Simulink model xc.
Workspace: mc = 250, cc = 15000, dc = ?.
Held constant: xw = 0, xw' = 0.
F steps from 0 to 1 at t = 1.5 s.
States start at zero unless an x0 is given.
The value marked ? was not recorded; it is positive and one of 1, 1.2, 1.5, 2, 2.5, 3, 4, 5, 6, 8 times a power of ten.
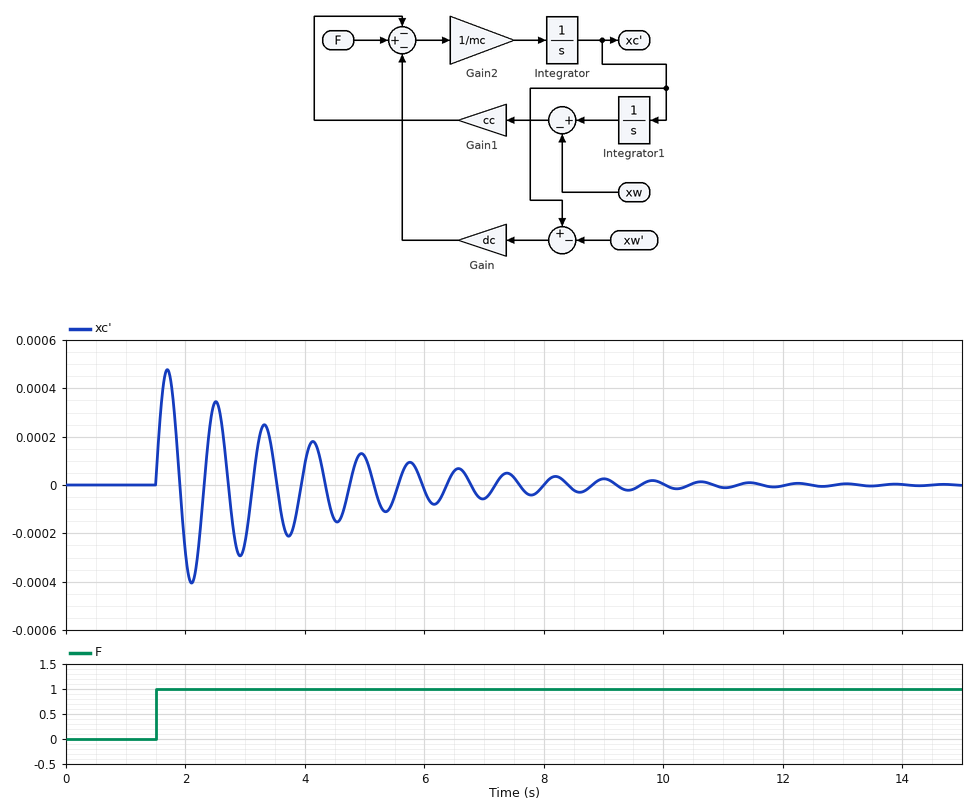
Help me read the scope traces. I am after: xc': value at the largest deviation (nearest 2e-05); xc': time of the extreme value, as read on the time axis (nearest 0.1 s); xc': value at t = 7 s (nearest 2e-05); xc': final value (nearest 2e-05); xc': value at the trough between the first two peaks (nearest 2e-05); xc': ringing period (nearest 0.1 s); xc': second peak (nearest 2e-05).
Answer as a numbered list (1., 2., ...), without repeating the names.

1. 0.00048
2. 1.7 s
3. -0.00006
4. 0.00000
5. -0.00040
6. 0.8 s
7. 0.00034
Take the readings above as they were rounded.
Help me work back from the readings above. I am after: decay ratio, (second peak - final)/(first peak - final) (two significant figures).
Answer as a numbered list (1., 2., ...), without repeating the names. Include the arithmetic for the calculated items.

1. (0.00034 - 0) / (0.00048 - 0) = 0.71
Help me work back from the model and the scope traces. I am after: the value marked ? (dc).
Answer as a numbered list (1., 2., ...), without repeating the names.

1. 200
